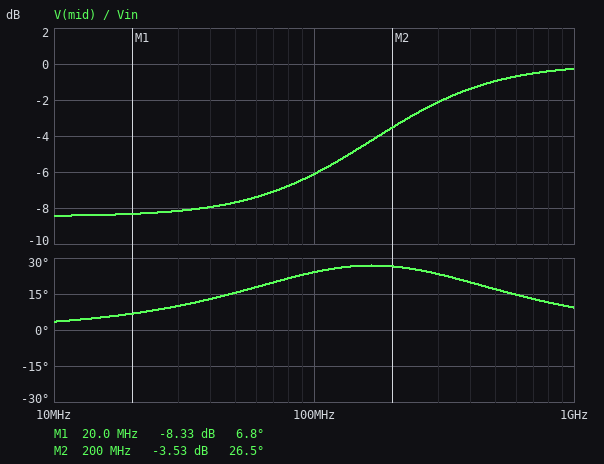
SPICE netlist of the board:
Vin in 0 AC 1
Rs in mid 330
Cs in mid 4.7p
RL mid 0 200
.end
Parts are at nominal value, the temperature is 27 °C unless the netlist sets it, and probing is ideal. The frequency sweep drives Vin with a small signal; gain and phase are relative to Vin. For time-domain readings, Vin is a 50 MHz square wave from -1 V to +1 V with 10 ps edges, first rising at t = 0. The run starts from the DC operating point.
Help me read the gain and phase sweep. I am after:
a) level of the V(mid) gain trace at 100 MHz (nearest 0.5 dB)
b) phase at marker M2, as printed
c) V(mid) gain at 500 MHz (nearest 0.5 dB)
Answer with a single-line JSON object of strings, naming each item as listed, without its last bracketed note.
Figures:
{"level of the V(mid) gain trace at 100 MHz": "-6.0 dB", "phase at marker M2, as printed": "26.5 deg", "V(mid) gain at 500 MHz": "-1.0 dB"}
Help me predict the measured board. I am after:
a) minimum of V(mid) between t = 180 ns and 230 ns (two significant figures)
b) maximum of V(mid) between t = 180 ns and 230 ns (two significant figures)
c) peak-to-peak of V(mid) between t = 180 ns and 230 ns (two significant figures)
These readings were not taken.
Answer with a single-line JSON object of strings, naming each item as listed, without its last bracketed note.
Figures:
{"minimum of V(mid) between t = 180 ns and 230 ns": "-1.6 V", "maximum of V(mid) between t = 180 ns and 230 ns": "1.6 V", "peak-to-peak of V(mid) between t = 180 ns and 230 ns": "3.2 V"}
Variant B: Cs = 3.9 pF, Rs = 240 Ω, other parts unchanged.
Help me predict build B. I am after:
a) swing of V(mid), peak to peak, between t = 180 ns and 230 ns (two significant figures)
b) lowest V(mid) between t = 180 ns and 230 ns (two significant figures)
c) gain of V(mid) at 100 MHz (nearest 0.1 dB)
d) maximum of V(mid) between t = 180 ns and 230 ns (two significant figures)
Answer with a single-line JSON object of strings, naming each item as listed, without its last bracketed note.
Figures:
{"swing of V(mid), peak to peak, between t = 180 ns and 230 ns": "3.1 V", "lowest V(mid) between t = 180 ns and 230 ns": "-1.5 V", "gain of V(mid) at 100 MHz": "-5.9 dB", "maximum of V(mid) between t = 180 ns and 230 ns": "1.5 V"}
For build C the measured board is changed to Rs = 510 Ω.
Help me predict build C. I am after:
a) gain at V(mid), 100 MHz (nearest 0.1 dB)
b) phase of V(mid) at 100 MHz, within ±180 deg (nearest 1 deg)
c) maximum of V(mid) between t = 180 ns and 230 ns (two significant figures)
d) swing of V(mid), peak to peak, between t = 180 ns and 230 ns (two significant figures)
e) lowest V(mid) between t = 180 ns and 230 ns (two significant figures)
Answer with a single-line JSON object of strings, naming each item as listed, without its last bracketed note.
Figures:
{"gain at V(mid), 100 MHz": "-6.6 dB", "phase of V(mid) at 100 MHz, within ±180 deg": "33 deg", "maximum of V(mid) between t = 180 ns and 230 ns": "1.7 V", "swing of V(mid), peak to peak, between t = 180 ns and 230 ns": "3.4 V", "lowest V(mid) between t = 180 ns and 230 ns": "-1.7 V"}
